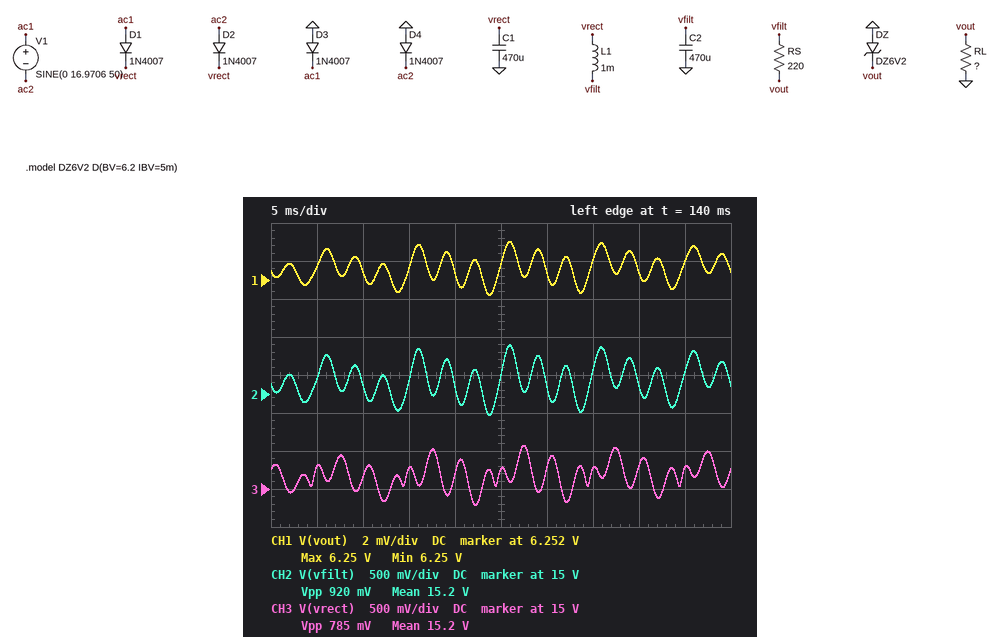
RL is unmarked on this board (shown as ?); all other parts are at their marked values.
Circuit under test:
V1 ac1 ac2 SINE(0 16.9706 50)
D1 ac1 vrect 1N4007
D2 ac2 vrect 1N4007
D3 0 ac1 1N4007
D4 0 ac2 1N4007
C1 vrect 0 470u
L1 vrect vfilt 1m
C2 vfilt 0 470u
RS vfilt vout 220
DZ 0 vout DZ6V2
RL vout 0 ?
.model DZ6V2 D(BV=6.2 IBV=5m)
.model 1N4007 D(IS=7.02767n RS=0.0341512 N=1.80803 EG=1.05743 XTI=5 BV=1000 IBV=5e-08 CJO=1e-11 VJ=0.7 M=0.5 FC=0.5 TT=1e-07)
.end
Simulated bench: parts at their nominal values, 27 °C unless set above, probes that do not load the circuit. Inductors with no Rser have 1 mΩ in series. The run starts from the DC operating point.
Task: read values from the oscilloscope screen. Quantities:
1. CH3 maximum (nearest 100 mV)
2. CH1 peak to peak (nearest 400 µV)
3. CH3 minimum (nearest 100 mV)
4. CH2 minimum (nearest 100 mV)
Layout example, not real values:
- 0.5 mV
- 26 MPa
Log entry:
- 15.6 V
- 2.8 mV
- 14.8 V
- 14.7 V
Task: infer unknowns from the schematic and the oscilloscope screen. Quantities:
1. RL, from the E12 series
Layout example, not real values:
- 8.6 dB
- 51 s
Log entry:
- 2.7 kΩ
